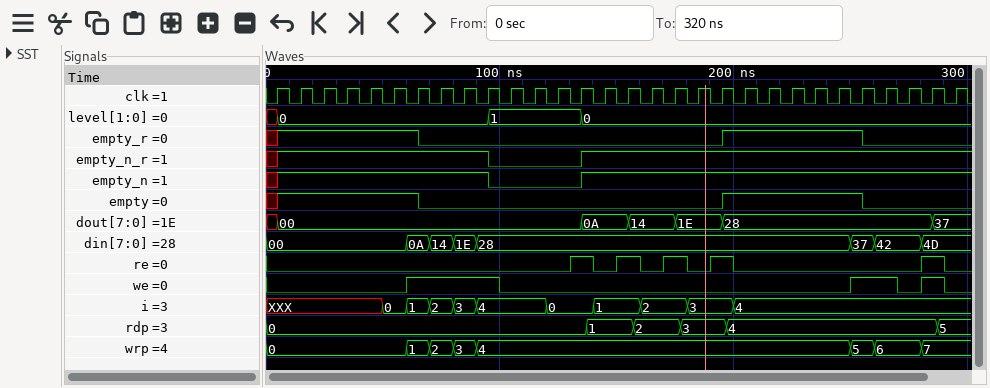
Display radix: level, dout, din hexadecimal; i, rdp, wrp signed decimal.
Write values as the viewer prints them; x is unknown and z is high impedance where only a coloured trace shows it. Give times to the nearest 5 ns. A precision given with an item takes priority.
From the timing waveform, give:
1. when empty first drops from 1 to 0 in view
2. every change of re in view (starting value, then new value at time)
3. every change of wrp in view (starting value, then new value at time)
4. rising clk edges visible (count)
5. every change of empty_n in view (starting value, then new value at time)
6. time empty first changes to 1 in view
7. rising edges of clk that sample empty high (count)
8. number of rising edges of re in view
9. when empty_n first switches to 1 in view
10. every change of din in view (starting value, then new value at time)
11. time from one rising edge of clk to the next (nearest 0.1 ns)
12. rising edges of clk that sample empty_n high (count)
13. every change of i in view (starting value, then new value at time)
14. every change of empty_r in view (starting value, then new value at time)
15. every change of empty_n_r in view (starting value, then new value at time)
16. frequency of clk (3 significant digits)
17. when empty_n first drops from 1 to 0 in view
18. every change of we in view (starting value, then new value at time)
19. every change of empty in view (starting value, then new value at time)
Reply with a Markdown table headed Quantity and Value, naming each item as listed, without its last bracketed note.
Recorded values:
| Quantity | Value |
|---|---|
| when empty first drops from 1 to 0 in view | 65 ns |
| every change of re in view | 0, 1 at 130 ns, 0 at 140 ns, 1 at 150 ns, 0 at 160 ns, 1 at 170 ns, 0 at 180 ns, 1 at 190 ns, 0 at 200 ns, 1 at 280 ns, 0 at 290 ns |
| every change of wrp in view | 0, 1 at 60 ns, 2 at 70 ns, 3 at 80 ns, 4 at 90 ns, 5 at 250 ns, 6 at 260 ns, 7 at 280 ns |
| rising clk edges visible | 30 |
| every change of empty_n in view | x, 1 at 5 ns, 0 at 95 ns, 1 at 135 ns |
| time empty first changes to 1 in view | 5 ns |
| rising edges of clk that sample empty high | 12 |
| number of rising edges of re in view | 5 |
| when empty_n first switches to 1 in view | 5 ns |
| every change of din in view | 00, 0A at 60 ns, 14 at 70 ns, 1E at 80 ns, 28 at 90 ns, 37 at 250 ns, 42 at 260 ns, 4D at 280 ns |
| time from one rising edge of clk to the next | 10 ns |
| rising edges of clk that sample empty_n high | 25 |
| every change of i in view | XXX, 0 at 50 ns, 1 at 60 ns, 2 at 70 ns, 3 at 80 ns, 4 at 90 ns, 0 at 120 ns, 1 at 140 ns, 2 at 160 ns, 3 at 180 ns, 4 at 200 ns |
| every change of empty_r in view | x, 1 at 5 ns, 0 at 65 ns, 1 at 195 ns, 0 at 255 ns |
| every change of empty_n_r in view | x, 1 at 5 ns, 0 at 95 ns, 1 at 135 ns |
| frequency of clk | 100 MHz |
| when empty_n first drops from 1 to 0 in view | 95 ns |
| every change of we in view | 0, 1 at 60 ns, 0 at 100 ns, 1 at 250 ns, 0 at 270 ns, 1 at 280 ns, 0 at 290 ns |
| every change of empty in view | x, 1 at 5 ns, 0 at 65 ns, 1 at 195 ns, 0 at 255 ns |
